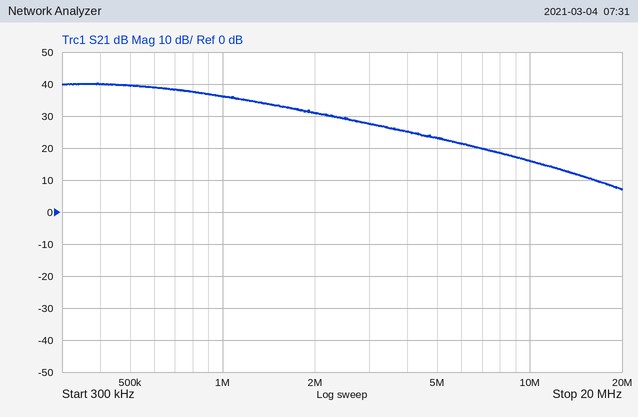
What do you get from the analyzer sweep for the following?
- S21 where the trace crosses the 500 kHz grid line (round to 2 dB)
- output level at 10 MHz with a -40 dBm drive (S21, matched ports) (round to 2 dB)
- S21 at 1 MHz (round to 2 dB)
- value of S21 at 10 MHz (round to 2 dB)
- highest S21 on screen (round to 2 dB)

40 dB
-24 dBm
36 dB
16 dB
40 dB
